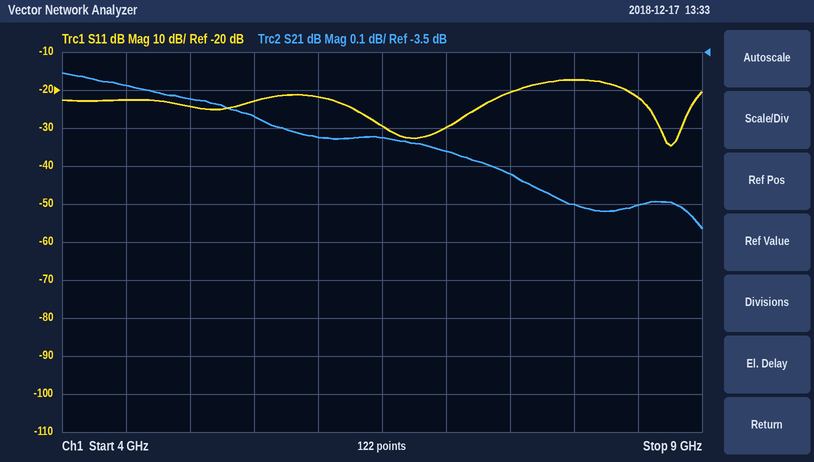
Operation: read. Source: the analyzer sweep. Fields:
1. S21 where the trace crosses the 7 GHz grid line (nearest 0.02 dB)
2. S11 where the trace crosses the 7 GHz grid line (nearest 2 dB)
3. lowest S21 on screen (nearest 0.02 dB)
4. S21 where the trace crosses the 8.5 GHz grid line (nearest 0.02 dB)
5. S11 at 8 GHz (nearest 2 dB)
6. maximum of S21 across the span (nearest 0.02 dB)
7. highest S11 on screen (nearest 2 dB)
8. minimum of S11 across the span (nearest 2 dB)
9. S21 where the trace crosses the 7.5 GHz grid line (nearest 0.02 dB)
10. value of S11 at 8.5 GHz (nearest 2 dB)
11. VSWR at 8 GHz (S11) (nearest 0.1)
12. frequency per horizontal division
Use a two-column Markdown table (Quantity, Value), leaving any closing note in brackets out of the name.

| Quantity | Value |
|---|---|
| S21 where the trace crosses the 7 GHz grid line | -3.76 dB |
| S11 where the trace crosses the 7 GHz grid line | -30 dB |
| lowest S21 on screen | -3.96 dB |
| S21 where the trace crosses the 8.5 GHz grid line | -3.90 dB |
| S11 at 8 GHz | -18 dB |
| maximum of S21 across the span | -3.56 dB |
| highest S11 on screen | -18 dB |
| minimum of S11 across the span | -34 dB |
| S21 where the trace crosses the 7.5 GHz grid line | -3.82 dB |
| value of S11 at 8.5 GHz | -22 dB |
| VSWR at 8 GHz (S11) | 1.3 |
| frequency per horizontal division | 500 MHz |
